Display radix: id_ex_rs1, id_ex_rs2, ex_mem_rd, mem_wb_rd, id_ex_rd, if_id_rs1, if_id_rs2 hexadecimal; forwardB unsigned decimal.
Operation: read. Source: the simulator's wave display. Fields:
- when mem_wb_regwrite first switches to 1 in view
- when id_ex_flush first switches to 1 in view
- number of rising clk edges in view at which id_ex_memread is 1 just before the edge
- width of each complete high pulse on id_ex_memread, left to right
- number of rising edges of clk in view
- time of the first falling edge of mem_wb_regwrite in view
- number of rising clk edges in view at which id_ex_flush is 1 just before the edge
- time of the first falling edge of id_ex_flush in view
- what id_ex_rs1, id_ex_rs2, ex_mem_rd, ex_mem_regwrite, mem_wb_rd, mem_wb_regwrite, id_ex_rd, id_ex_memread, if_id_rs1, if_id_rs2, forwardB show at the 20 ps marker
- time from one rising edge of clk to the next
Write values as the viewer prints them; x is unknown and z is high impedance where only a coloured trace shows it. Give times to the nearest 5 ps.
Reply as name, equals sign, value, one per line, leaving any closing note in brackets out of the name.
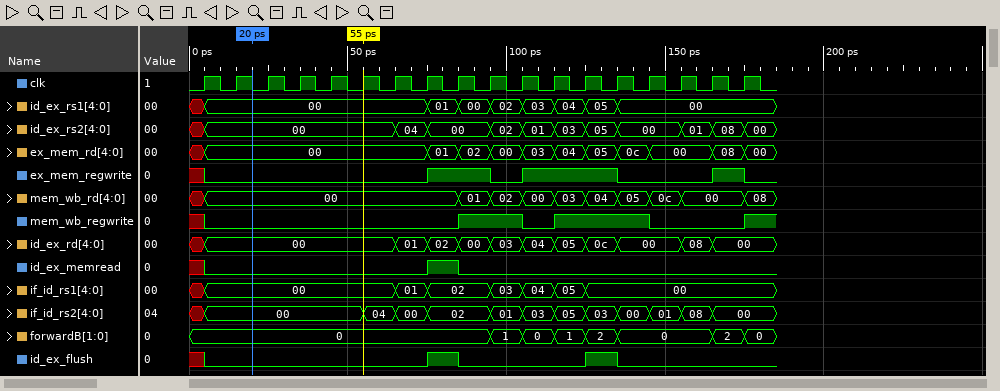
when mem_wb_regwrite first switches to 1 in view = 85 ps
when id_ex_flush first switches to 1 in view = 75 ps
number of rising clk edges in view at which id_ex_memread is 1 just before the edge = 1
width of each complete high pulse on id_ex_memread, left to right = 10 ps
number of rising edges of clk in view = 18
time of the first falling edge of mem_wb_regwrite in view = 105 ps
number of rising clk edges in view at which id_ex_flush is 1 just before the edge = 2
time of the first falling edge of id_ex_flush in view = 85 ps
what id_ex_rs1, id_ex_rs2, ex_mem_rd, ex_mem_regwrite, mem_wb_rd, mem_wb_regwrite, id_ex_rd, id_ex_memread, if_id_rs1, if_id_rs2, forwardB show at the 20 ps marker = id_ex_rs1=00, id_ex_rs2=00, ex_mem_rd=00, ex_mem_regwrite=0, mem_wb_rd=00, mem_wb_regwrite=0, id_ex_rd=00, id_ex_memread=0, if_id_rs1=00, if_id_rs2=00, forwardB=0
time from one rising edge of clk to the next = 10 ps
